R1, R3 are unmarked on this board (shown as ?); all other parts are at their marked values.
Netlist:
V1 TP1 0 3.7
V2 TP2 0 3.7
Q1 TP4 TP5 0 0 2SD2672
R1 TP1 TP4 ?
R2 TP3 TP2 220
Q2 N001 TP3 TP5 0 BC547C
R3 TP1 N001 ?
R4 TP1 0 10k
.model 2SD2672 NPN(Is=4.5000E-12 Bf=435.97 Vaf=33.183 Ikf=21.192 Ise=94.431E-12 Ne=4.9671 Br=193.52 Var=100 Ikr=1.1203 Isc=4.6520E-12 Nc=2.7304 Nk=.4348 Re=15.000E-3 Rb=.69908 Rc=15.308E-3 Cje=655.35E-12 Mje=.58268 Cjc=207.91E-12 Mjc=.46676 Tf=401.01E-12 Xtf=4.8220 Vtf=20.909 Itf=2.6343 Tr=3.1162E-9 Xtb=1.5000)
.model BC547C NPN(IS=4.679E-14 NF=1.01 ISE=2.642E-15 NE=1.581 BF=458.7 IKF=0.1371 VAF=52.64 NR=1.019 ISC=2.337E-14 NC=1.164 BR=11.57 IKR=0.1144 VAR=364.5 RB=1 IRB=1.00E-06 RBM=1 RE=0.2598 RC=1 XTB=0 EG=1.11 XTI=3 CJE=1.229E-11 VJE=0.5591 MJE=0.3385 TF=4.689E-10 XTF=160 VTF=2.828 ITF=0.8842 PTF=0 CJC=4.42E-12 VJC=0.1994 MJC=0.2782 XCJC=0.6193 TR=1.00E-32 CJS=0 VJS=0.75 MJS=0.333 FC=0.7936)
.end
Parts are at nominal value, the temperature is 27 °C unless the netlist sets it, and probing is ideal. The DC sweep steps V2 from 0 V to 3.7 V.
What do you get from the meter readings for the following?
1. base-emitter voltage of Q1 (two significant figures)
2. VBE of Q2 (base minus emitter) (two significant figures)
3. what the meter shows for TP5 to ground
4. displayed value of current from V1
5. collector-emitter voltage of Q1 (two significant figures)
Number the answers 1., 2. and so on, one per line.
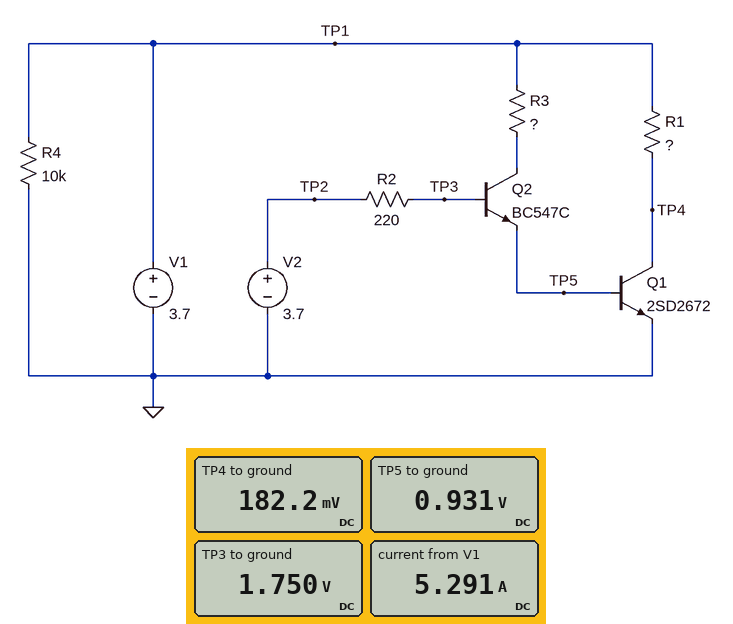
1. 930 mV
2. 820 mV
3. 0.931 V
4. 5.291 A
5. 180 mV
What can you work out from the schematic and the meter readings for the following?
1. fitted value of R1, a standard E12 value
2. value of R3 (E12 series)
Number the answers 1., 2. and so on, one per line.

1. 0.68 Ω
2. 22 Ω
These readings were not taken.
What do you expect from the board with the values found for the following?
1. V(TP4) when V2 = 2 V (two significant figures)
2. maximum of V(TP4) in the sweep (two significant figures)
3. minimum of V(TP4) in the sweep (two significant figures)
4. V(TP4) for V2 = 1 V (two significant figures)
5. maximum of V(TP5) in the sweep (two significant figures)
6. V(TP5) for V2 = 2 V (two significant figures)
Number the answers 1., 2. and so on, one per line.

1. 180 mV
2. 3.7 V
3. 180 mV
4. 3.7 V
5. 930 mV
6. 920 mV
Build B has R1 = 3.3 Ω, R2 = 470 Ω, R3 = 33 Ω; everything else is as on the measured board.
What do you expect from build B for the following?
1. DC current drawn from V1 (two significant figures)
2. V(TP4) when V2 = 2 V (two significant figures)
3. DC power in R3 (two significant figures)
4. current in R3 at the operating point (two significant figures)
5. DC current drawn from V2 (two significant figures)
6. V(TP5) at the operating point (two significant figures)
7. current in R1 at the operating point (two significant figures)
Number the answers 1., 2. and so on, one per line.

1. 1.2 A
2. 43 mV
3. 230 mW
4. 83 mA
5. 4.4 mA
6. 820 mV
7. 1.1 A
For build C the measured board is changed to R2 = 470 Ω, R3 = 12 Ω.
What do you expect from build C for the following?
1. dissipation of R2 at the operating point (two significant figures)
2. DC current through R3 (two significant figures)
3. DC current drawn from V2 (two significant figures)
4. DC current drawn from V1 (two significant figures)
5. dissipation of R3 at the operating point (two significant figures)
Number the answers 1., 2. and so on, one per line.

1. 7.4 mW
2. 200 mA
3. 4.0 mA
4. 5.4 A
5. 470 mW
